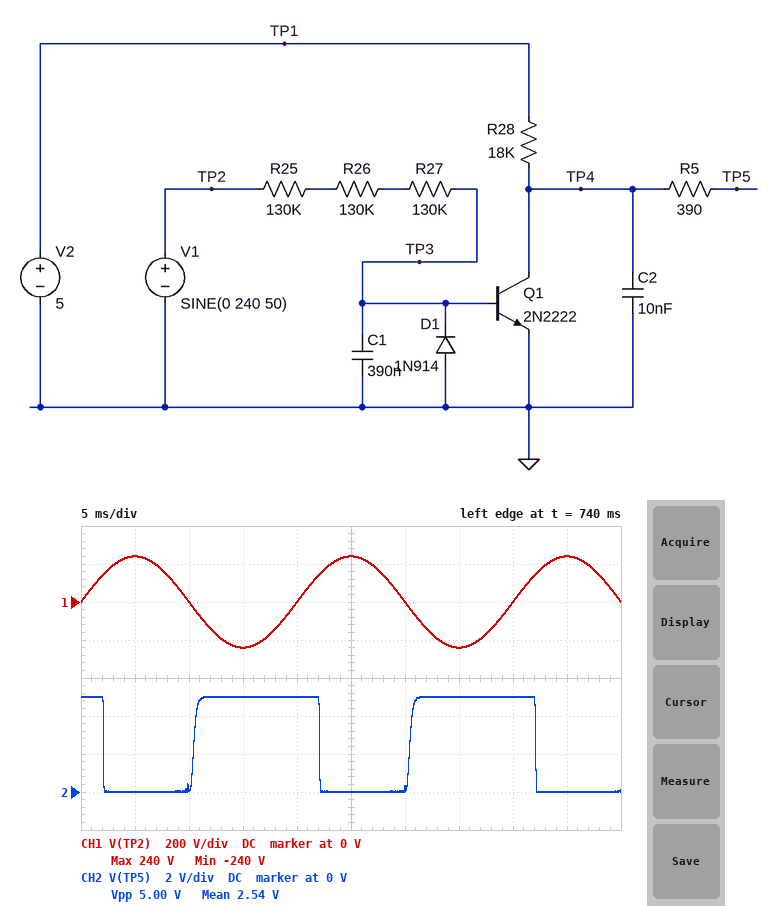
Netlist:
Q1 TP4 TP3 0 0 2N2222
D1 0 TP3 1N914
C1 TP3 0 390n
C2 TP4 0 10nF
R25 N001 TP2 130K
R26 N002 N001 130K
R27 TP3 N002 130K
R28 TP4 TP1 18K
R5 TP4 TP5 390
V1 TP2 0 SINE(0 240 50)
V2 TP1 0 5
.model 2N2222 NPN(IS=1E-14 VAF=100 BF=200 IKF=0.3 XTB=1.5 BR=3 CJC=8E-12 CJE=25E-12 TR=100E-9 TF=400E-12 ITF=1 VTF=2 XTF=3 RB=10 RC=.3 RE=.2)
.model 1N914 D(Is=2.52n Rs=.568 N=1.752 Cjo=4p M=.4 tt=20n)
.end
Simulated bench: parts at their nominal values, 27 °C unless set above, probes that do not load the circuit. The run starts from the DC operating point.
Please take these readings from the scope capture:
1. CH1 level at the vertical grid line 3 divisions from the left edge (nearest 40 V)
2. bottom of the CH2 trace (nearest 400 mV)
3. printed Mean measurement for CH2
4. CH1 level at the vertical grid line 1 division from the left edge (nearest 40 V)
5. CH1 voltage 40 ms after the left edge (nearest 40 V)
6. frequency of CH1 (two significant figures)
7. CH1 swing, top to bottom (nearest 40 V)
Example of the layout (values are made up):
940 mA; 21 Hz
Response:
-240 V; 0 V; 2.54 V; 240 V; 0 V; 50 Hz; 480 V
